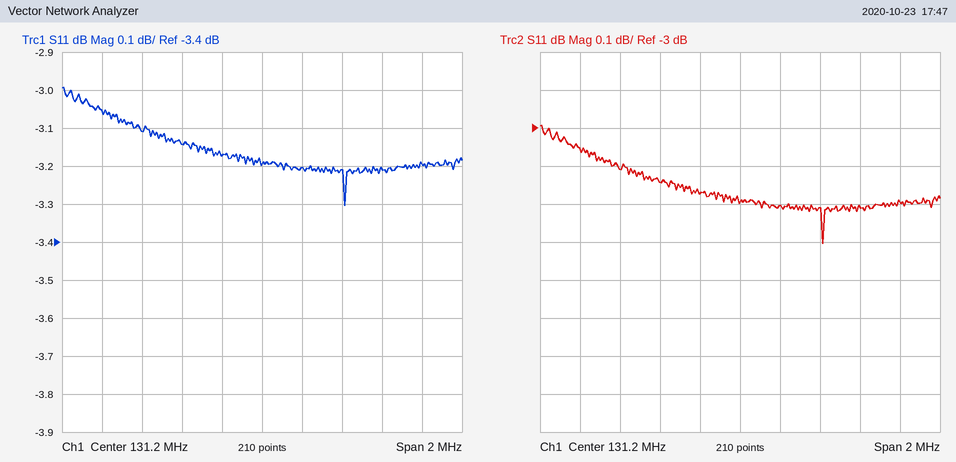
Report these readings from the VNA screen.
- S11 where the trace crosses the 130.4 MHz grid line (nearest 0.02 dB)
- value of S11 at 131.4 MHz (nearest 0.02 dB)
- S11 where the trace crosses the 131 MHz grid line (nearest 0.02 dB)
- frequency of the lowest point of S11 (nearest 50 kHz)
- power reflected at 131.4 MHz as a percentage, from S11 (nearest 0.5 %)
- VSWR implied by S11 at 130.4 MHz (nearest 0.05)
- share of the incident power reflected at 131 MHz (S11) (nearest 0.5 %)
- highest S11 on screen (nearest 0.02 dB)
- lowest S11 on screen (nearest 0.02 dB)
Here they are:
-3.06 dB
-3.20 dB
-3.18 dB
131.60 MHz
48.0 %
5.75
48.0 %
-3.00 dB
-3.30 dB
